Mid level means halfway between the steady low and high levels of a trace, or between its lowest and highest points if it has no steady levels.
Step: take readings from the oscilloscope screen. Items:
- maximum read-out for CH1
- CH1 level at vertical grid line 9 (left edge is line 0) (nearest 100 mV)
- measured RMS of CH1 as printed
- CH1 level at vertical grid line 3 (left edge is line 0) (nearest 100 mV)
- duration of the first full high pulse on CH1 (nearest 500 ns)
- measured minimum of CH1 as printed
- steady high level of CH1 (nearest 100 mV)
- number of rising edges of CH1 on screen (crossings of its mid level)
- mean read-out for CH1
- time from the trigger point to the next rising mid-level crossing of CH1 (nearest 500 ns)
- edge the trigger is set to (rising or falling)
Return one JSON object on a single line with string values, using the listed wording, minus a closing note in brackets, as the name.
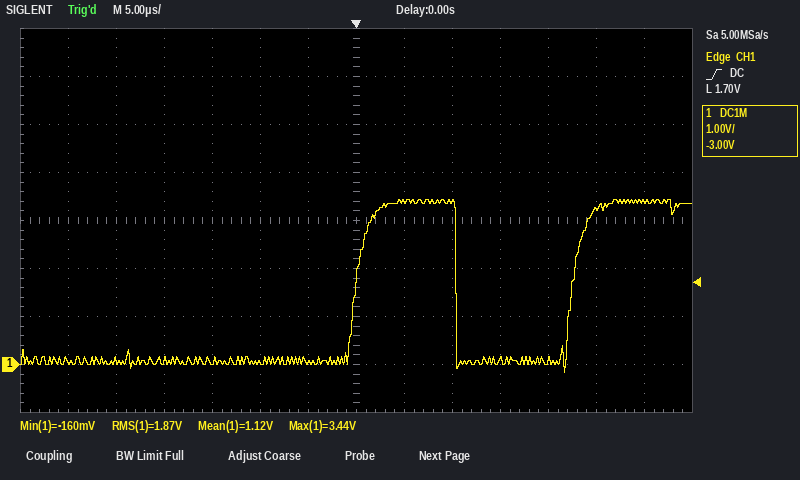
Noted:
{"maximum read-out for CH1": "3.44 V", "CH1 level at vertical grid line 9 (left edge is line 0)": "3.4 V", "measured RMS of CH1 as printed": "1.87 V", "CH1 level at vertical grid line 3 (left edge is line 0)": "100 mV", "duration of the first full high pulse on CH1": "10.5 µs", "measured minimum of CH1 as printed": "-160 mV", "steady high level of CH1": "3.4 V", "number of rising edges of CH1 on screen": "2", "mean read-out for CH1": "1.12 V", "time from the trigger point to the next rising mid-level crossing of CH1": "22.5 µs", "edge the trigger is set to": "rising"}
